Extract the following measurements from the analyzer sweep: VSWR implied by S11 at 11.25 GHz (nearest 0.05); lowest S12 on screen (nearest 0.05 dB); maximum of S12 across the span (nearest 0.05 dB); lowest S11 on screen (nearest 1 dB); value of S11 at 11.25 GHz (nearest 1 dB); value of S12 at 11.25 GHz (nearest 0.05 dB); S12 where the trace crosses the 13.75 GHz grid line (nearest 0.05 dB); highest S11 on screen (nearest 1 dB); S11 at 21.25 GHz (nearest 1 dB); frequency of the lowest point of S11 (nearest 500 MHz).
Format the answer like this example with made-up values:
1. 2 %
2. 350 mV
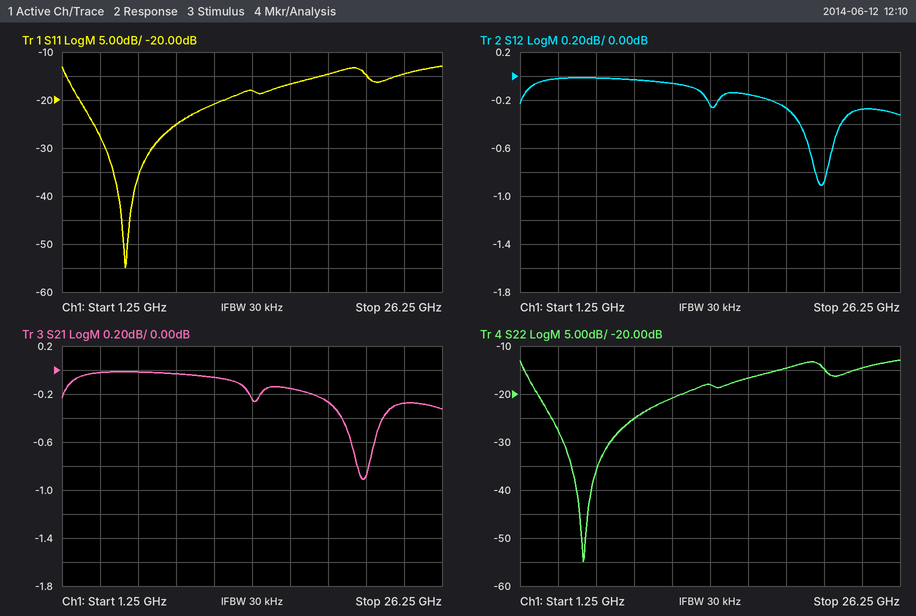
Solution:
1. 1.20
2. -0.90 dB
3. 0.00 dB
4. -55 dB
5. -21 dB
6. -0.05 dB
7. -0.25 dB
8. -13 dB
9. -15 dB
10. 5.5 GHz
